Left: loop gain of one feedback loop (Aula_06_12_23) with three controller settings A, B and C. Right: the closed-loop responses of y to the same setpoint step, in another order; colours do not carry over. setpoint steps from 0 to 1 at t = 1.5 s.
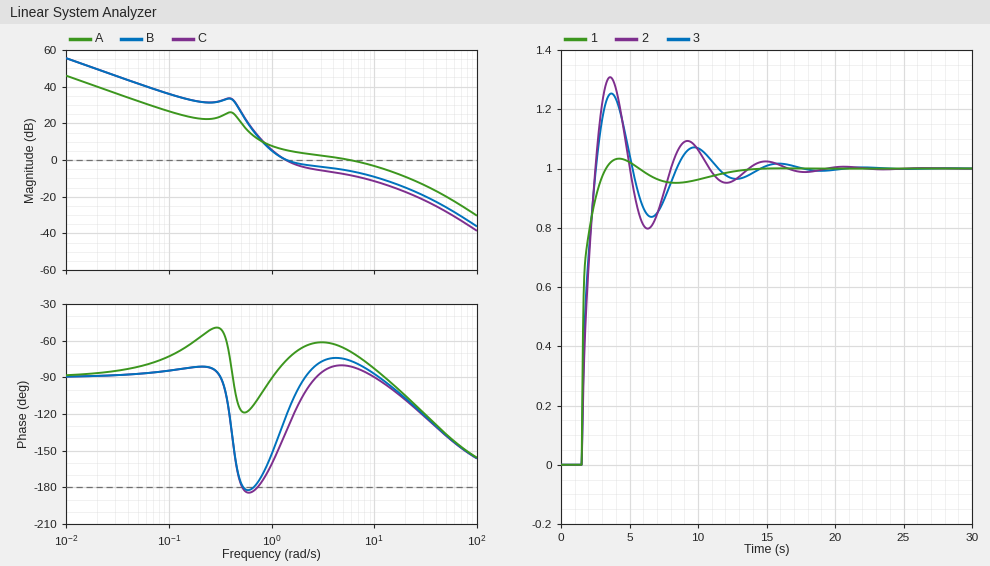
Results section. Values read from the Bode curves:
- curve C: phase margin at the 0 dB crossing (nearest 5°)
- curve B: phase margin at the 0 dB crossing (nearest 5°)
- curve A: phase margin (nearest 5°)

45°
60°
110°
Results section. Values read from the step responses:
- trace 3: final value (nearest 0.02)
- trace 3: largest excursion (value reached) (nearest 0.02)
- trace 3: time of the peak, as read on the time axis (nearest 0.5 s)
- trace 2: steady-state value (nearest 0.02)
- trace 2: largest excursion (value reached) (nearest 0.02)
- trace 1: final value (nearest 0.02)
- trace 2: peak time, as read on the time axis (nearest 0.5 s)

1.00
1.26
3.5 s
1.00
1.30
1.00
3.5 s
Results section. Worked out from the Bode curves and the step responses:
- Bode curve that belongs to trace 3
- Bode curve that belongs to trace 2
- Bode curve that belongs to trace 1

B
C
A
